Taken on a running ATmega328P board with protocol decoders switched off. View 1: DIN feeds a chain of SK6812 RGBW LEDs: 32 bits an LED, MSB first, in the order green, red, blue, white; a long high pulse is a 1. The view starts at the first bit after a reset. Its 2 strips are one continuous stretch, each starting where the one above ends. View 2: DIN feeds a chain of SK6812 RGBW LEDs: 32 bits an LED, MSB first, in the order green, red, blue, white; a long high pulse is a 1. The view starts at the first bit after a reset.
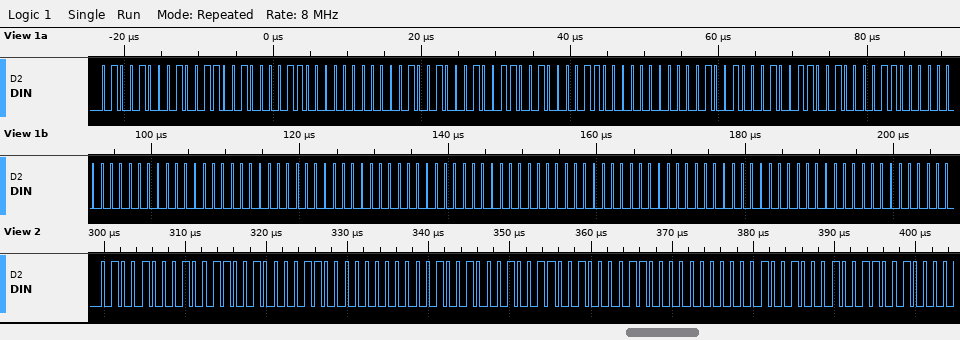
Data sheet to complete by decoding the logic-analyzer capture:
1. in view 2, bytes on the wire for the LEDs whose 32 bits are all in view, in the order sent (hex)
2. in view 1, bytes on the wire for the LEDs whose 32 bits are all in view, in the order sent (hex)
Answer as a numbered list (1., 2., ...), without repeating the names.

1. 48 99 0C 00 48 99 0C 00
2. 48 99 0C 00 48 99 0C 00 48 99 0C 00 00 00 00 00 00 00 00 00
